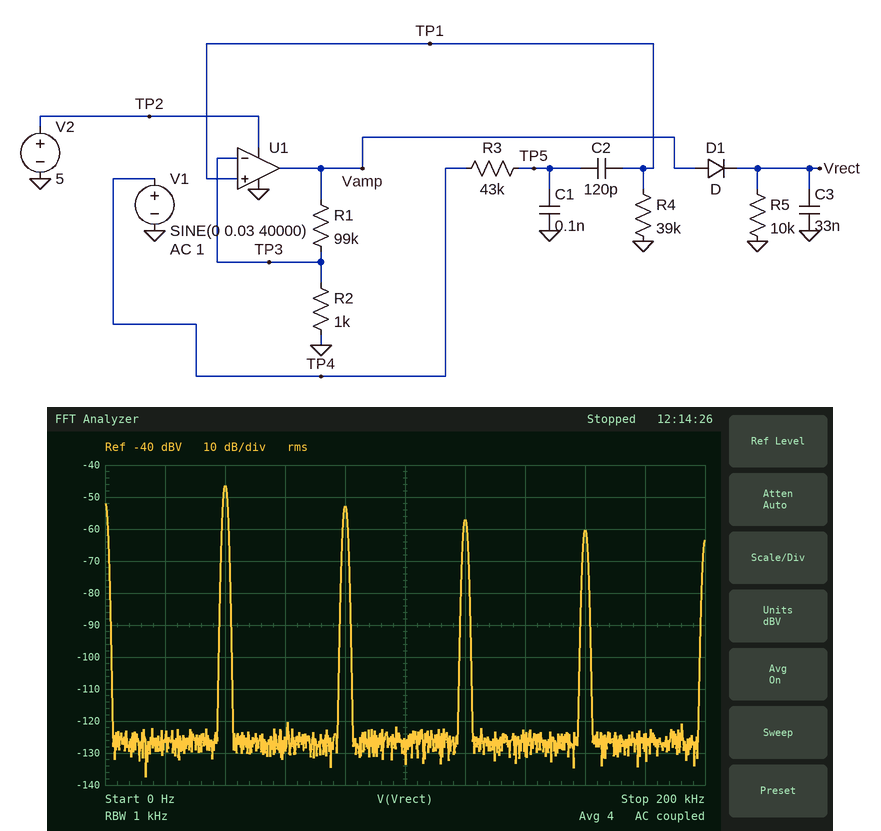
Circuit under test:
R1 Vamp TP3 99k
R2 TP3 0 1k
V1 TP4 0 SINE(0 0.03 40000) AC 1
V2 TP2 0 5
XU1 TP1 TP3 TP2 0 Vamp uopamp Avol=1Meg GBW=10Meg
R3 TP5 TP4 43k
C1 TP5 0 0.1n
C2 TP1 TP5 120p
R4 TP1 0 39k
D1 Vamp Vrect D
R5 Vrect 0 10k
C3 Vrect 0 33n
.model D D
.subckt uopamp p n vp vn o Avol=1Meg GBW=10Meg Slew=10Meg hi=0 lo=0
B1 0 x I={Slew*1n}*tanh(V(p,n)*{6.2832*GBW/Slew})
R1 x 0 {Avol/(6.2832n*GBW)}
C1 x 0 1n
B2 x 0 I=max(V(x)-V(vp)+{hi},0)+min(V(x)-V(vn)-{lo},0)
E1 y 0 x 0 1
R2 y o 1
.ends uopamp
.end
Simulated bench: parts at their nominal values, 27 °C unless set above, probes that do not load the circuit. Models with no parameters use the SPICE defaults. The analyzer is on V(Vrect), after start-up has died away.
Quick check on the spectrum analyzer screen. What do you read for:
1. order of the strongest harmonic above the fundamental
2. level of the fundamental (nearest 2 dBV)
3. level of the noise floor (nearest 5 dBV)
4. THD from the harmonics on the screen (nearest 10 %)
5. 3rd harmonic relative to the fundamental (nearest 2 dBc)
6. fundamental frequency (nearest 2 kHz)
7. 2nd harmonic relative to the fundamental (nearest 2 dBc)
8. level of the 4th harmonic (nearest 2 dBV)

2
-46 dBV
-125 dBV
60 %
-10 dBc
40 kHz
-6 dBc
-60 dBV
